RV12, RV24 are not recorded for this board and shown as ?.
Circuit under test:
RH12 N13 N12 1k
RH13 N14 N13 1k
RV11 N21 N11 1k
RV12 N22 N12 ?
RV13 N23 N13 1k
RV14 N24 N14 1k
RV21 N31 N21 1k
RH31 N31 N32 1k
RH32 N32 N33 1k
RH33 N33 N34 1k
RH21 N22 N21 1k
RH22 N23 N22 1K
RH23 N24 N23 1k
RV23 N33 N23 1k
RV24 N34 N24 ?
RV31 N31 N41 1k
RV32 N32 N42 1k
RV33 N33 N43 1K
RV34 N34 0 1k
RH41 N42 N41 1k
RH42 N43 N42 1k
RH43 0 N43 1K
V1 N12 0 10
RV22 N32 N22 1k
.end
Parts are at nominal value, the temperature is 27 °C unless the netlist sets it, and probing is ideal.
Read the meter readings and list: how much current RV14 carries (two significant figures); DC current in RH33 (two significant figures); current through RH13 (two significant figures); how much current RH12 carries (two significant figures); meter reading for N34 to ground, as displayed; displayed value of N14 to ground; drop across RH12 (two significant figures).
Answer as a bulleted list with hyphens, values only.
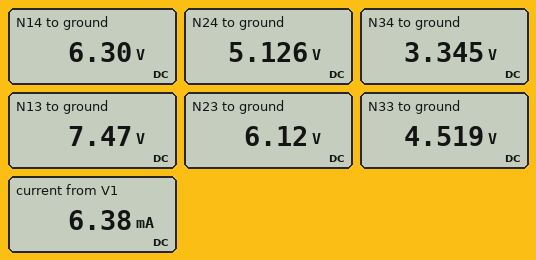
- 1.2 mA
- 1.2 mA
- 1.2 mA
- 2.5 mA
- 3.345 V
- 6.30 V
- 2.5 V
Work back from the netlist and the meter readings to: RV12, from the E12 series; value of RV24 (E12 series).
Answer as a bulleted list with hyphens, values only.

- 680 Ω
- 820 Ω
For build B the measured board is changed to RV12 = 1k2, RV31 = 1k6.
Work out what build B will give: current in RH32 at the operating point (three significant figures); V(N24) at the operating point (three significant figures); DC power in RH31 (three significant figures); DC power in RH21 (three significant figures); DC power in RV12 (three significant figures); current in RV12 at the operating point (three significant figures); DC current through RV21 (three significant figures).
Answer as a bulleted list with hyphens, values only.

- 840 µA
- 4.77 V
- 48.1 µW
- 419 µW
- 10.6 mW
- 2.97 mA
- 648 µA
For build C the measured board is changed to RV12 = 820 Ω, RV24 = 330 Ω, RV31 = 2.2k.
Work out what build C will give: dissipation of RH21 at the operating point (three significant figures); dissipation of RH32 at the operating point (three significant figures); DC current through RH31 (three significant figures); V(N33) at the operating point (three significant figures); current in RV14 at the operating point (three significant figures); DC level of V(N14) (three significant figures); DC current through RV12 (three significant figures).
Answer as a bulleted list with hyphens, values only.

- 484 µW
- 909 µW
- 288 µA
- 4.39 V
- 1.38 mA
- 5.81 V
- 3.64 mA
